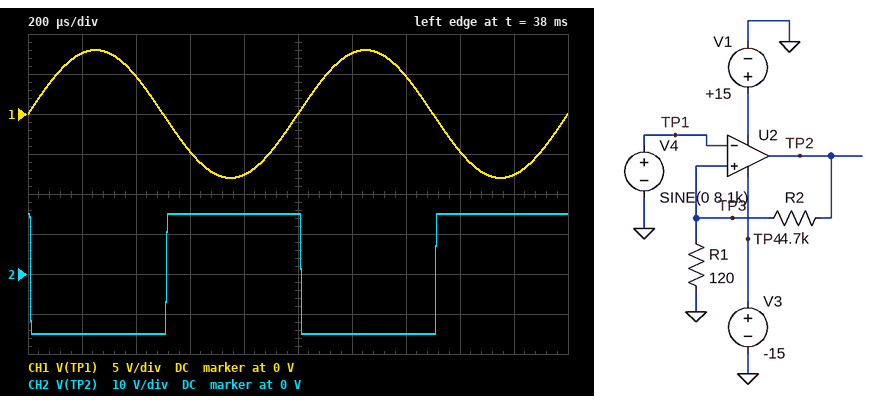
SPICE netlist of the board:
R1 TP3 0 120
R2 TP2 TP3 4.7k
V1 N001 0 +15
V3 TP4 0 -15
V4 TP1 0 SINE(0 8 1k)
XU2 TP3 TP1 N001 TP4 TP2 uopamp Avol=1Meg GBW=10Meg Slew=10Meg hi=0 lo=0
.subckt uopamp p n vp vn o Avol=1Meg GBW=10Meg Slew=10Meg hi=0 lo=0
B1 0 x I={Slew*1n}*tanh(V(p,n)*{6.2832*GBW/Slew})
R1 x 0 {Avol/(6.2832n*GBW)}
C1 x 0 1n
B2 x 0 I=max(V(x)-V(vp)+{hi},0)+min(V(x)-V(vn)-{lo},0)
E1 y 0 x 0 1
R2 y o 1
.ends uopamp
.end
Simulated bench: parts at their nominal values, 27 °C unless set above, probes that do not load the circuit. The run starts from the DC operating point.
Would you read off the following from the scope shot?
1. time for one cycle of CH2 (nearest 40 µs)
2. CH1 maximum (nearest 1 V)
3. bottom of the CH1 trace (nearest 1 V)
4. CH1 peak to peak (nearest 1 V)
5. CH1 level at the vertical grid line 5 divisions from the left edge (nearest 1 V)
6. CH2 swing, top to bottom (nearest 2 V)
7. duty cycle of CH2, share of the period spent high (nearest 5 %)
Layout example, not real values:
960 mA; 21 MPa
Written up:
1.00 ms; 8 V; -8 V; 16 V; 0 V; 30 V; 50 %
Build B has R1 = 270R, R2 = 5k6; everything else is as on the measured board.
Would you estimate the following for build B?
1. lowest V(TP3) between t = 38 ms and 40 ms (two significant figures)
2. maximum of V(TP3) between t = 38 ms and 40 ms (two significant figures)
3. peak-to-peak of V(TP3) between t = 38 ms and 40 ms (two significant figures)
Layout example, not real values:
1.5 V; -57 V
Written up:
-690 mV; 690 mV; 1.4 V
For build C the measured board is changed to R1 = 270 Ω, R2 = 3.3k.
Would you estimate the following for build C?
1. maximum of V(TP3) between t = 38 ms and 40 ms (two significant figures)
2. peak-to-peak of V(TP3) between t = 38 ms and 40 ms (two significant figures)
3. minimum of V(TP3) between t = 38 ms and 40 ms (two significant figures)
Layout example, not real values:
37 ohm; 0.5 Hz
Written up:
1.1 V; 2.3 V; -1.1 V
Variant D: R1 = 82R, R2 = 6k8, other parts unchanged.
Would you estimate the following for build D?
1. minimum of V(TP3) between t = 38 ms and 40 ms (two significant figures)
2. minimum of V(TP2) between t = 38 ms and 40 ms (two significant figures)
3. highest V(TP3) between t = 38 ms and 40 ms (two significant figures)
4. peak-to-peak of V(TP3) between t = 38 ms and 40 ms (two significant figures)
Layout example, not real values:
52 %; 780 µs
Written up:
-180 mV; -15 V; 180 mV; 360 mV
